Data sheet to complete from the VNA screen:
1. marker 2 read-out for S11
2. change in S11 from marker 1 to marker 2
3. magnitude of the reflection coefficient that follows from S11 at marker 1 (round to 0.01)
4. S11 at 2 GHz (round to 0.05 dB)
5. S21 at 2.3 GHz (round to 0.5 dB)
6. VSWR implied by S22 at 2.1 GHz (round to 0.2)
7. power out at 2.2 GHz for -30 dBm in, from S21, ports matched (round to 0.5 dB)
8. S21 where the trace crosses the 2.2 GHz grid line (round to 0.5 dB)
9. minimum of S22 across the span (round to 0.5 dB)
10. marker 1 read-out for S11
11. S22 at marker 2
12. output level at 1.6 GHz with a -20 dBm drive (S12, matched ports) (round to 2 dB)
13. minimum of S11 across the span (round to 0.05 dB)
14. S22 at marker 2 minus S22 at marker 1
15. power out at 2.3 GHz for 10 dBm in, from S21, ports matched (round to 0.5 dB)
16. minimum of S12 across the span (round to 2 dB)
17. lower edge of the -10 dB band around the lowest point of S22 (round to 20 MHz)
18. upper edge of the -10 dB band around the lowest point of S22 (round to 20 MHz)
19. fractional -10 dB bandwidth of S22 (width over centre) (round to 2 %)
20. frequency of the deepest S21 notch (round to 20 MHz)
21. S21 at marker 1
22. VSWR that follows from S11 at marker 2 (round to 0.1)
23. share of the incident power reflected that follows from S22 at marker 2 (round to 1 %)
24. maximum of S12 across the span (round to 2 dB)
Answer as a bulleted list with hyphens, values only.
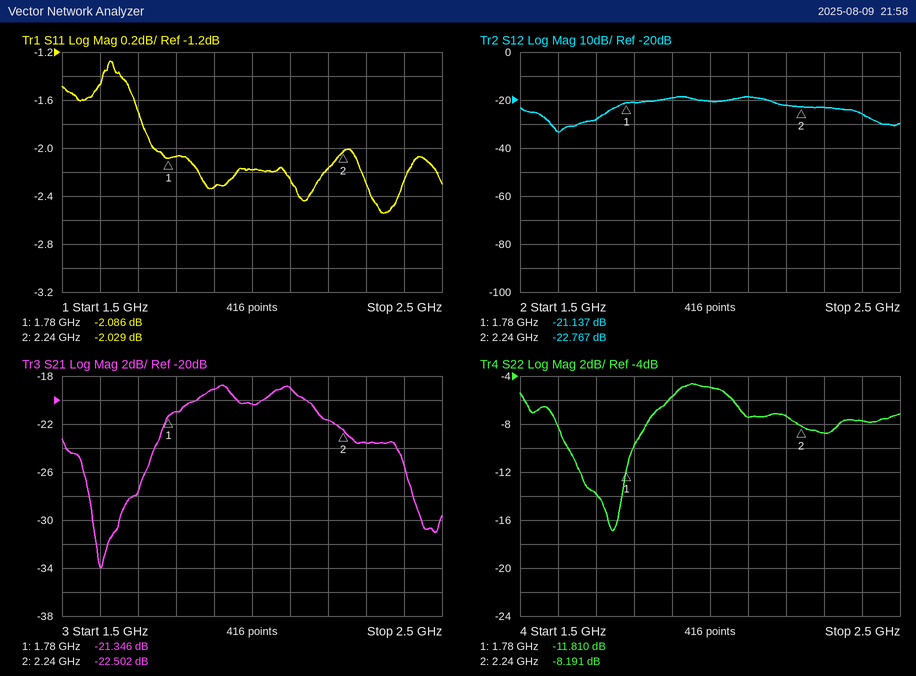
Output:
- -2.029 dB
- 0.057 dB
- 0.79
- -2.20 dB
- -23.5 dB
- 2.4
- -51.5 dBm
- -21.5 dB
- -17.0 dB
- -2.086 dB
- -8.191 dB
- -54 dBm
- -2.55 dB
- 3.619 dB
- -13.5 dBm
- -34 dB
- 1.62 GHz
- 1.80 GHz
- 10 %
- 1.60 GHz
- -21.346 dB
- 8.6
- 15 %
- -18 dB
